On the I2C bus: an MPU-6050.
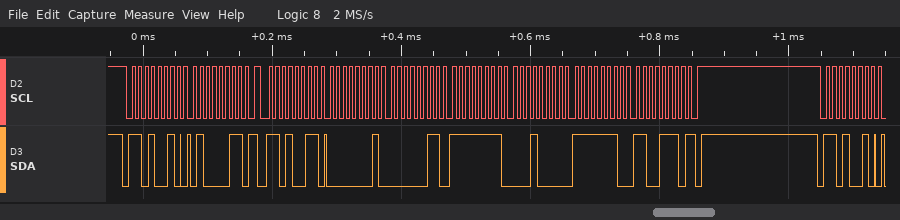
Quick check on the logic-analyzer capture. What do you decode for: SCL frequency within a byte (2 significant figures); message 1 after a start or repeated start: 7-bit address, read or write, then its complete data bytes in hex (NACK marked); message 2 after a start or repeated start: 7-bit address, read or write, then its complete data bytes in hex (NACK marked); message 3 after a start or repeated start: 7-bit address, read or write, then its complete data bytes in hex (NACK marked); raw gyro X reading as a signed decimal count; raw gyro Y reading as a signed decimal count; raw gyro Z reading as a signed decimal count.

100 kHz
0x69 write: 43
0x69 read: 01 03 FF 10 FE CE NACK
0x69 write
259
-240
-306
